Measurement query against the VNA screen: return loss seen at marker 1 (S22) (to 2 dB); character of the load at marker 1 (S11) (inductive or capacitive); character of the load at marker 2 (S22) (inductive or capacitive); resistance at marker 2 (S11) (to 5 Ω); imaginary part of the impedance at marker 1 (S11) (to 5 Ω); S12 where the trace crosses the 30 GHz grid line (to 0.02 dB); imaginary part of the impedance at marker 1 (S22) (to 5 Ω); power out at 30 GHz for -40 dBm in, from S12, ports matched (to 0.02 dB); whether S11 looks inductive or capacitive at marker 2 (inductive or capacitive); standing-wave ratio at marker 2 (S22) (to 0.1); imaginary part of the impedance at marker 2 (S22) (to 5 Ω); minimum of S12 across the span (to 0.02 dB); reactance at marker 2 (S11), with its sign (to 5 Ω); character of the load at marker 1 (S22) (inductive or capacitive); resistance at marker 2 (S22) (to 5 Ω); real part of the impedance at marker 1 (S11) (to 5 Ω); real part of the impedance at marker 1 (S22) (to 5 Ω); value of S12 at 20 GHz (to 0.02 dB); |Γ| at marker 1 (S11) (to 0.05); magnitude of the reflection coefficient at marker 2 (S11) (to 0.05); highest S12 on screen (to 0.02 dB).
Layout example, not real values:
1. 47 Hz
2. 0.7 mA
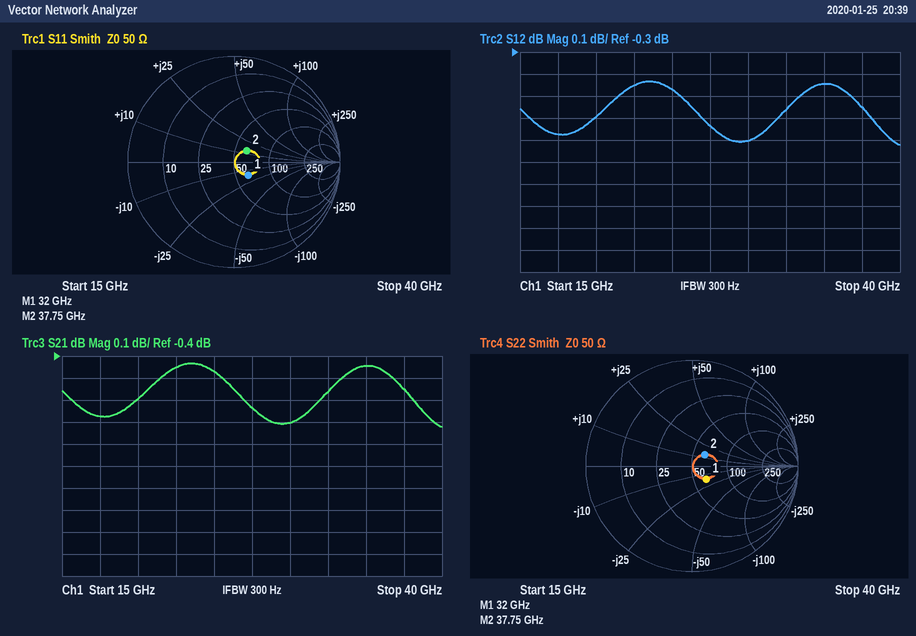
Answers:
1. 14 dB
2. capacitive
3. inductive
4. 60 Ω
5. -15 Ω
6. -0.70 dB
7. -15 Ω
8. -40.70 dBm
9. inductive
10. 1.4
11. +15 Ω
12. -0.72 dB
13. +15 Ω
14. capacitive
15. 60 Ω
16. 65 Ω
17. 65 Ω
18. -0.60 dB
19. 0.20
20. 0.15
21. -0.44 dB
